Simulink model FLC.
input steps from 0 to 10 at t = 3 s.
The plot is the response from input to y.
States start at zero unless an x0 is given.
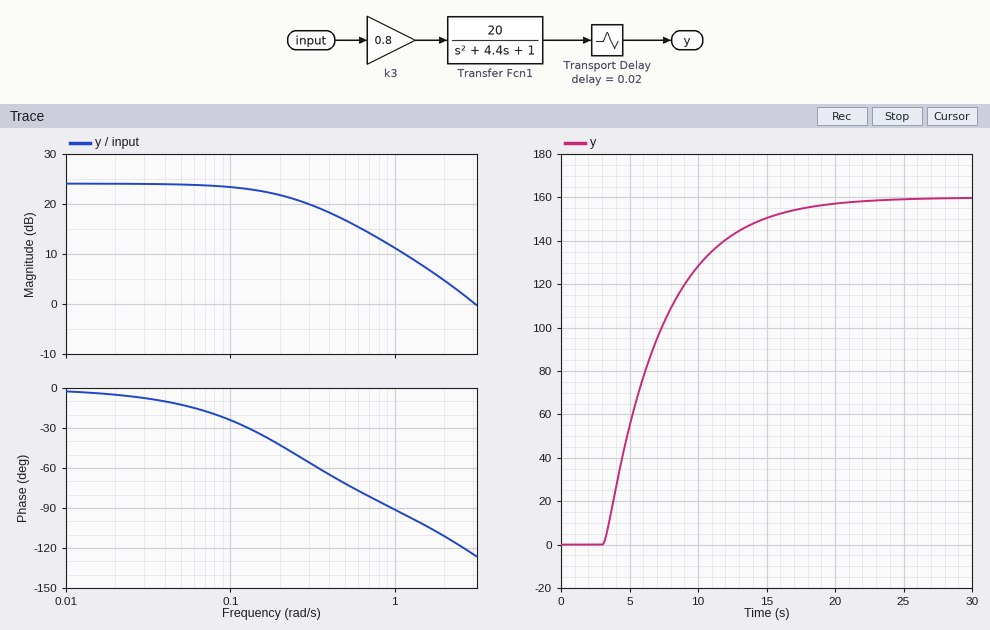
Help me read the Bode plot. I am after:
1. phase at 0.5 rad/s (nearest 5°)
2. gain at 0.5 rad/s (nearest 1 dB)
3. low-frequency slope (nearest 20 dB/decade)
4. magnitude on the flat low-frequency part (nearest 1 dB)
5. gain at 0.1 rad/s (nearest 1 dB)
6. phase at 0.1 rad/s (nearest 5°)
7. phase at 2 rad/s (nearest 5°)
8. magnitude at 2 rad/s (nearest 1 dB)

-70°
17 dB
0 dB/decade
24 dB
23 dB
-25°
-110°
5 dB
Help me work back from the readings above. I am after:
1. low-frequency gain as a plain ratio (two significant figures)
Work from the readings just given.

16
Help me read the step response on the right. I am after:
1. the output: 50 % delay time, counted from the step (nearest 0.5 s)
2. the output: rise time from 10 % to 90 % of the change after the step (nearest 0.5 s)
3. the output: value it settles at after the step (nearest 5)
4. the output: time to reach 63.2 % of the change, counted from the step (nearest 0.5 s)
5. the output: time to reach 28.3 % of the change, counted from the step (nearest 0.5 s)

3.0 s
9.0 s
160
4.5 s
1.5 s
